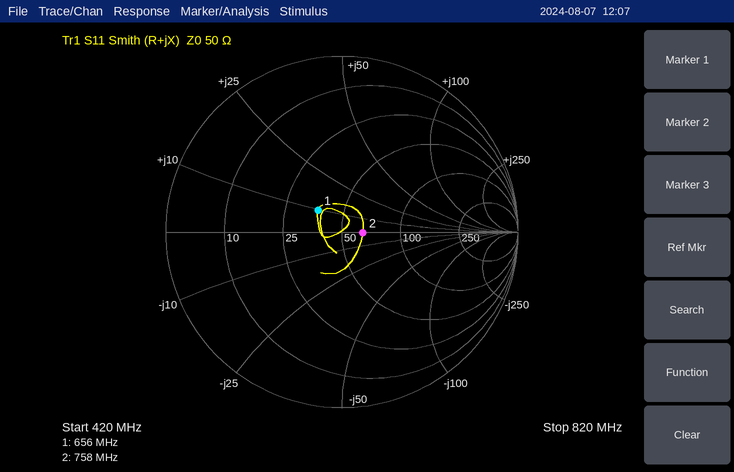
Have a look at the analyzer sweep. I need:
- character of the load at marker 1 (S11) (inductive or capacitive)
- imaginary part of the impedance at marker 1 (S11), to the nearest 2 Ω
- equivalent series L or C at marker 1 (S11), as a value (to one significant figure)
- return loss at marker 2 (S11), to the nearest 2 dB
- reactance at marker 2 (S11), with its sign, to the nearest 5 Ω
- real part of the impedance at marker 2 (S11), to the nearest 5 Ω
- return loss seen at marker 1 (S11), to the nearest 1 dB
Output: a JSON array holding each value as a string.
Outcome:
["inductive", "+10 Ω", "2 nH", "18 dB", "0 Ω", "65 Ω", "15 dB"]
